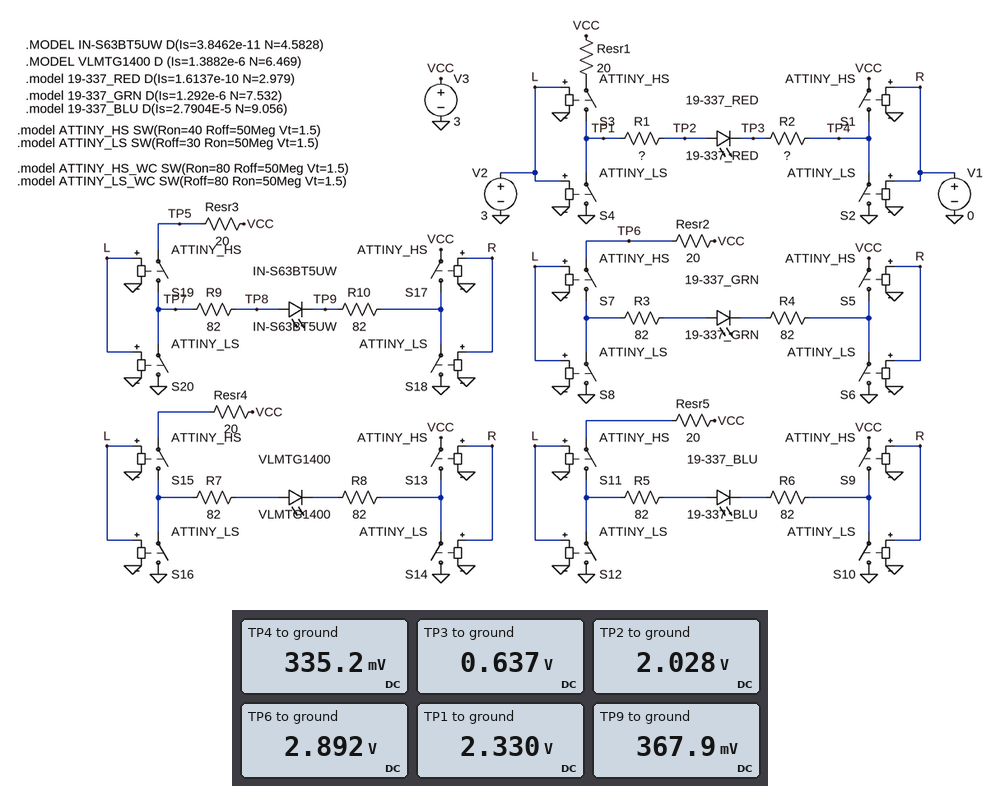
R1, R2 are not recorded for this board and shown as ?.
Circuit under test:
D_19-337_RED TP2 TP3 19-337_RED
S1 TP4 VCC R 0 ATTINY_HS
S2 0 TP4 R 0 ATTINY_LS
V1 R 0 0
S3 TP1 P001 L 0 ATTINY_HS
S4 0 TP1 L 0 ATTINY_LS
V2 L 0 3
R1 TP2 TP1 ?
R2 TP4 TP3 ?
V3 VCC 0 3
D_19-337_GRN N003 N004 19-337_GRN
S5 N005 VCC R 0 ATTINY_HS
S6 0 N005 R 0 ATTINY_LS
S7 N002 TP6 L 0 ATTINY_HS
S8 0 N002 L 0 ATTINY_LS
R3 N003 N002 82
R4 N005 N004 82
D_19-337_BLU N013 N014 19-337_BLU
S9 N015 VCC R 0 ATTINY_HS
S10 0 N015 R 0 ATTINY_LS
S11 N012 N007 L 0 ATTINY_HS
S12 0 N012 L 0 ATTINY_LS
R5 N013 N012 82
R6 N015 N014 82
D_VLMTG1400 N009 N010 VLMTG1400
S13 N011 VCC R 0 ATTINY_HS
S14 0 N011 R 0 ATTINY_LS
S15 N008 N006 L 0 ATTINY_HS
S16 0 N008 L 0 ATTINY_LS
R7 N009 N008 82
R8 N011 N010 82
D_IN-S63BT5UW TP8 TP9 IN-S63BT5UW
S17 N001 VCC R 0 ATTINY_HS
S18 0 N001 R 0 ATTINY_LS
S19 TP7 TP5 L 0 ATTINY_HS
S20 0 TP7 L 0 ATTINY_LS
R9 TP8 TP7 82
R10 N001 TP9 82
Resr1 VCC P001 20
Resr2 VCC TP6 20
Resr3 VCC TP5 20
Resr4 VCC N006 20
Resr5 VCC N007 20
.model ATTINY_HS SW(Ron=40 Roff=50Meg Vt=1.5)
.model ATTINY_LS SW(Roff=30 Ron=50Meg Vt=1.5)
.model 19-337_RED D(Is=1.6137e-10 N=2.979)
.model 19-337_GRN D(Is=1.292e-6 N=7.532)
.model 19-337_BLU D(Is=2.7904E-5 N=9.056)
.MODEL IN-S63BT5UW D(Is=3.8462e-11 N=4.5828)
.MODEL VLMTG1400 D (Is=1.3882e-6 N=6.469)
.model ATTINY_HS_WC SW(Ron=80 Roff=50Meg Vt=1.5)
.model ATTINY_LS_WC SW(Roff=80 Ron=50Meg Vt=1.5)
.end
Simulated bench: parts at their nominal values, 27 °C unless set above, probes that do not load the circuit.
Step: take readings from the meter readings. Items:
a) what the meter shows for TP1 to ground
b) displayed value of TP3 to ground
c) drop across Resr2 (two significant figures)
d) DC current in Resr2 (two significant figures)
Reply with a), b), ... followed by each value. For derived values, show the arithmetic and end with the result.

a) 2.330 V
b) 0.637 V
c) 3 V - 2.892 V = 110 mV
d) (3 V - 2.892 V) / 20 Ω = 5.4 mA
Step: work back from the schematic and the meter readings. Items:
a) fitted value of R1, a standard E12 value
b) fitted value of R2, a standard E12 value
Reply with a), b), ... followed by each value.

a) 27 Ω
b) 27 Ω
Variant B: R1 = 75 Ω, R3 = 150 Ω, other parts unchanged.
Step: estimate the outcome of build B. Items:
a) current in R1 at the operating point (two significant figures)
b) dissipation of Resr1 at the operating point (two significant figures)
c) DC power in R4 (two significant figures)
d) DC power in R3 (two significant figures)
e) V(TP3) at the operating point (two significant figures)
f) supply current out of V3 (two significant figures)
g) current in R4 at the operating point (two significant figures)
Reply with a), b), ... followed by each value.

a) 8.5 mA
b) 1.4 mW
c) 1.6 mW
d) 2.9 mW
e) 480 mV
f) 29 mA
g) 4.4 mA
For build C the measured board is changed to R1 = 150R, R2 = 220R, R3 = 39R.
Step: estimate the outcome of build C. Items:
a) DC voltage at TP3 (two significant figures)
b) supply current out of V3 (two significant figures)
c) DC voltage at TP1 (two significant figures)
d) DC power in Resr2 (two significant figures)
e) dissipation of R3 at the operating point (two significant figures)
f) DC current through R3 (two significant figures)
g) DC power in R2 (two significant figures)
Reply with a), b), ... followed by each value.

a) 920 mV
b) 26 mA
c) 2.8 V
d) 810 µW
e) 1.6 mW
f) 6.4 mA
g) 3.0 mW
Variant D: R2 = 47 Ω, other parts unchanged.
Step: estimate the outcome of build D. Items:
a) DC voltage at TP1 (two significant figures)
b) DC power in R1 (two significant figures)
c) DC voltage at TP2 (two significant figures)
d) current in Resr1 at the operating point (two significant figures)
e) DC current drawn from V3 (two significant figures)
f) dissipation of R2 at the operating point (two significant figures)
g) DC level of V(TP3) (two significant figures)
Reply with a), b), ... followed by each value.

a) 2.4 V
b) 2.6 mW
c) 2.1 V
d) 9.9 mA
e) 32 mA
f) 4.6 mW
g) 760 mV
